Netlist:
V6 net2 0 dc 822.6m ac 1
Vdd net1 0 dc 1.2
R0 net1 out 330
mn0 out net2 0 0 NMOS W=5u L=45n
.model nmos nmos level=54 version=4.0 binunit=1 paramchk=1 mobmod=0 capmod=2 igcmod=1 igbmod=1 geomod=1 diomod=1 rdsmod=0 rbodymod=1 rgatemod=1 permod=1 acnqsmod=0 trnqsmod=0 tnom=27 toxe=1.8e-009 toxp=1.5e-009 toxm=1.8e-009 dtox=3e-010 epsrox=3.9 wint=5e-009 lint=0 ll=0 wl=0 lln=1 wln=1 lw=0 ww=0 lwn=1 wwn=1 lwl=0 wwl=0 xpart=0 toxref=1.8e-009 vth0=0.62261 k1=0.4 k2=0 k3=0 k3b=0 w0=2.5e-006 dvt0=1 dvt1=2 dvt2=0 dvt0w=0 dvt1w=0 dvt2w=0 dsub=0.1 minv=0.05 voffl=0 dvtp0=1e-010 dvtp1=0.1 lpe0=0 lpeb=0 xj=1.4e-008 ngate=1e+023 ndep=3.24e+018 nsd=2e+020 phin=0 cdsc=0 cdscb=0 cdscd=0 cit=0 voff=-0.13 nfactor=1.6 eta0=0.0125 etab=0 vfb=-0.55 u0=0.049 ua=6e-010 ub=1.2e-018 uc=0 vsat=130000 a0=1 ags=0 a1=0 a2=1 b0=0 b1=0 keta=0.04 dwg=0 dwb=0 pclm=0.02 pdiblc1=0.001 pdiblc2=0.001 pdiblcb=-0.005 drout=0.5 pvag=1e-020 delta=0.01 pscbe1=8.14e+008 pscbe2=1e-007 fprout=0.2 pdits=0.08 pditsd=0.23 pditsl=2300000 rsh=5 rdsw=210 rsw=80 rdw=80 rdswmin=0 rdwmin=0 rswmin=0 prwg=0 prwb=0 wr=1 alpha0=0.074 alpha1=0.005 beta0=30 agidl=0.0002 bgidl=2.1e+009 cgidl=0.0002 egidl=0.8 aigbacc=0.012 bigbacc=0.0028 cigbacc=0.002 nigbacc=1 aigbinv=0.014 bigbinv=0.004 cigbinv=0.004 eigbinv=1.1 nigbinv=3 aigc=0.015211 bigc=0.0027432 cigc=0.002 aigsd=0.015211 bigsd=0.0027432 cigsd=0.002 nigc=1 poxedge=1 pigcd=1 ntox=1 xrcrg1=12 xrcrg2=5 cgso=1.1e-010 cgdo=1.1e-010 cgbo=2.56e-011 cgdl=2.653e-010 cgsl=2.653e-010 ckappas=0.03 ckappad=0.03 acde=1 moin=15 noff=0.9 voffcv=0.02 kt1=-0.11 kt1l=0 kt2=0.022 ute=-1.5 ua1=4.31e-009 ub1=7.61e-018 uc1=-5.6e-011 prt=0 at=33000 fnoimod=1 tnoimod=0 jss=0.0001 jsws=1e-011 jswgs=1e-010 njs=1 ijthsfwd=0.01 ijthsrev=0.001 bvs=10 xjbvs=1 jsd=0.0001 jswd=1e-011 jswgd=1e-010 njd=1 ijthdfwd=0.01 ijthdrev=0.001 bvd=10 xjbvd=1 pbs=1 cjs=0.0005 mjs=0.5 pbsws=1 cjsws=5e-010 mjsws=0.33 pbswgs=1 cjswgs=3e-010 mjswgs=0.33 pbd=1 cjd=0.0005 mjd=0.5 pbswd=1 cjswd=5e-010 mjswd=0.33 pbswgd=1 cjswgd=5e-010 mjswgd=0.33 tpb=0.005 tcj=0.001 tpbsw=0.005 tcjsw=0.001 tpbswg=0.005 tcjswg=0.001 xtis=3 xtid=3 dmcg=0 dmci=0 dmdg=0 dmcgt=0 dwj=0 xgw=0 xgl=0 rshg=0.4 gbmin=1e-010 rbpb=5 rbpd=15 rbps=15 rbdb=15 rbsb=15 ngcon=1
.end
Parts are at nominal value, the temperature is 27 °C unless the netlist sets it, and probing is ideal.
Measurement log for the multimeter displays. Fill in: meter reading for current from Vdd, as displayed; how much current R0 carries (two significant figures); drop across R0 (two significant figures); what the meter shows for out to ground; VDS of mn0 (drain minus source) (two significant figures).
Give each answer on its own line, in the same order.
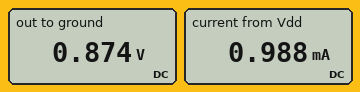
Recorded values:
0.988 mA
990 µA
330 mV
0.874 V
870 mV
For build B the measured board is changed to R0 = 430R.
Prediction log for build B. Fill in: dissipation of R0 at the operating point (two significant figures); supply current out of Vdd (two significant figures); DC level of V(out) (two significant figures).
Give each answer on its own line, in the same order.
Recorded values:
390 µW
950 µA
790 mV
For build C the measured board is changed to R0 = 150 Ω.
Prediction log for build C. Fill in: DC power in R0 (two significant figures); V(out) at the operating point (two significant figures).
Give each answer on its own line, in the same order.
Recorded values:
170 µW
1.0 V
